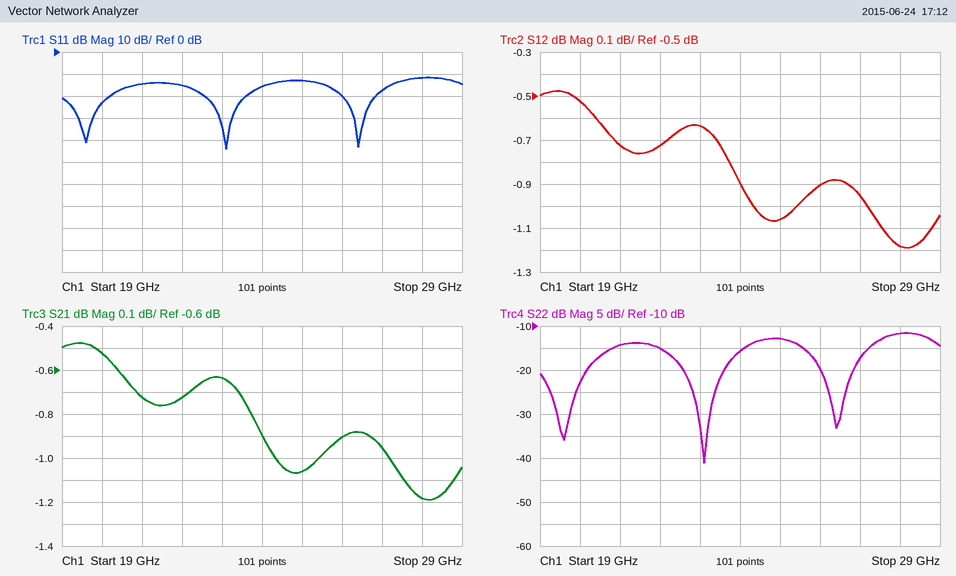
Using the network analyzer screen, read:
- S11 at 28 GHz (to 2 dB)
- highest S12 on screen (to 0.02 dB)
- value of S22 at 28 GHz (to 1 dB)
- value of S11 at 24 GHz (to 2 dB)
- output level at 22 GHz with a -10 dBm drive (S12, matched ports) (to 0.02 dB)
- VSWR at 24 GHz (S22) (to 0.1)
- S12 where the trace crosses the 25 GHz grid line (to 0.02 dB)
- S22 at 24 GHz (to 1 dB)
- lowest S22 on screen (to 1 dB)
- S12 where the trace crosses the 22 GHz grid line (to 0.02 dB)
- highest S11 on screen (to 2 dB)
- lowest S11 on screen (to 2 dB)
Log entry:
-12 dB
-0.48 dB
-12 dB
-16 dB
-10.72 dBm
1.4
-1.06 dB
-16 dB
-41 dB
-0.72 dB
-12 dB
-44 dB
